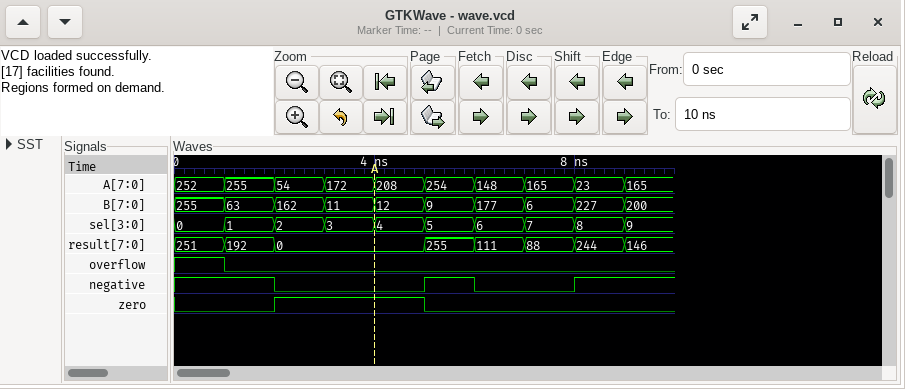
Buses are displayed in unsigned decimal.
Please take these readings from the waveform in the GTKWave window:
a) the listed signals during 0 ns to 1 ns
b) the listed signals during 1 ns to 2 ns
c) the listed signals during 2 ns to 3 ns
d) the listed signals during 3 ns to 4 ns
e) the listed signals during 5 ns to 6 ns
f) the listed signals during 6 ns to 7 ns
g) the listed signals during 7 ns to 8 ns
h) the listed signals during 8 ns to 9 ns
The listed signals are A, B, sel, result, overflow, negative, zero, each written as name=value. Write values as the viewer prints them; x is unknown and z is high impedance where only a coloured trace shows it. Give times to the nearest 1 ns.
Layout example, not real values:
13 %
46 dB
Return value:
A=252, B=255, sel=0, result=251, overflow=1, negative=1, zero=0
A=255, B=63, sel=1, result=192, overflow=0, negative=1, zero=0
A=54, B=162, sel=2, result=0, overflow=0, negative=0, zero=1
A=172, B=11, sel=3, result=0, overflow=0, negative=0, zero=1
A=254, B=9, sel=5, result=255, overflow=0, negative=1, zero=0
A=148, B=177, sel=6, result=111, overflow=0, negative=0, zero=0
A=165, B=6, sel=7, result=88, overflow=0, negative=0, zero=0
A=23, B=227, sel=8, result=244, overflow=0, negative=1, zero=0
